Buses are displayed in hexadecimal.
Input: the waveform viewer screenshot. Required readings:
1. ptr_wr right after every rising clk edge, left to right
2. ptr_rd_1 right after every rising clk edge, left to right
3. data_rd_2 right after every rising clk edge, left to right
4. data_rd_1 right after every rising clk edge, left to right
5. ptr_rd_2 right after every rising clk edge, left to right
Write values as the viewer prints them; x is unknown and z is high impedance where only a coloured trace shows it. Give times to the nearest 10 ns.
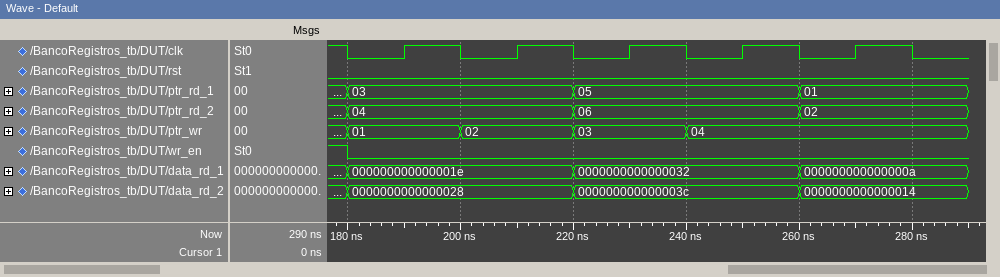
01, 02, 03, 04, 04
03, 03, 05, 05, 01
0000000000000028, 0000000000000028, 000000000000003c, 000000000000003c, 0000000000000014
000000000000001e, 000000000000001e, 0000000000000032, 0000000000000032, 000000000000000a
04, 04, 06, 06, 02
